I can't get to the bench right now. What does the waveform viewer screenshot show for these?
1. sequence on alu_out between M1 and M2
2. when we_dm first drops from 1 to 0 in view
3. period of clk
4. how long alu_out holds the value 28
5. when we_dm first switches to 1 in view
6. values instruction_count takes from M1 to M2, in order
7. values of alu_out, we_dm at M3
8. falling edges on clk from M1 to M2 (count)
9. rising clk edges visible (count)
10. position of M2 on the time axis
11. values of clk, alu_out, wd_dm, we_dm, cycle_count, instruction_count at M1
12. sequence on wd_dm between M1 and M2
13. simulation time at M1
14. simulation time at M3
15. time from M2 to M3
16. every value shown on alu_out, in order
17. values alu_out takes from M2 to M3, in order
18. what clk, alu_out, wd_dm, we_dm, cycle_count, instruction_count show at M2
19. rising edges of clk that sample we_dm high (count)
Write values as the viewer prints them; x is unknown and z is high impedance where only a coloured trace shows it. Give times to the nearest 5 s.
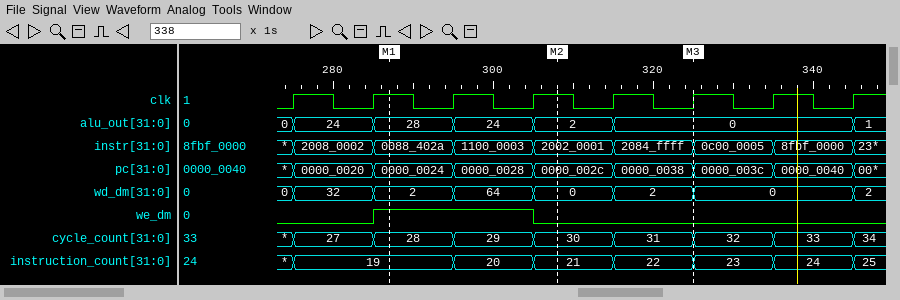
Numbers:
28, 24, 2
305 s
10 s
10 s
285 s
19, 20, 21
alu_out=0, we_dm=0
2
8
310 s
clk=1, alu_out=28, wd_dm=2, we_dm=1, cycle_count=28, instruction_count=19
2, 64, 0
285 s
325 s
15 s
0, 24, 28, 24, 2, 0, 1
2, 0
clk=1, alu_out=2, wd_dm=0, we_dm=0, cycle_count=30, instruction_count=21
2
